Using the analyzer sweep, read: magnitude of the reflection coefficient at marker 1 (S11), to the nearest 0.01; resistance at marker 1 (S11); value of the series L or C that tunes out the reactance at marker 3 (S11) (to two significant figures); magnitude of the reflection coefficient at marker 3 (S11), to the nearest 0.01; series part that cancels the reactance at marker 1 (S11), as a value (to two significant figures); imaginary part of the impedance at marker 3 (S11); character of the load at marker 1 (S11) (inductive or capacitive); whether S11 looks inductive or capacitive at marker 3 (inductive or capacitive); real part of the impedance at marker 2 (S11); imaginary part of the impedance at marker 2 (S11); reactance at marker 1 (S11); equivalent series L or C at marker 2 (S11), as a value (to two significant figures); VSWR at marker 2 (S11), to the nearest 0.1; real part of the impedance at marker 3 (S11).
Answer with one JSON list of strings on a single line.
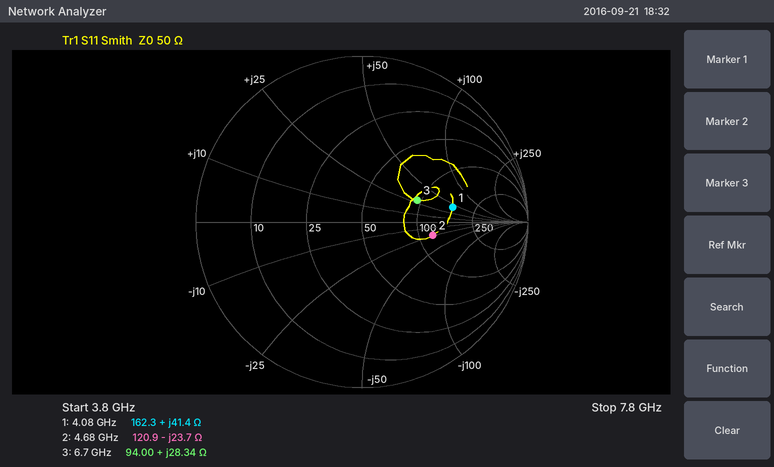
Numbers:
["0.55", "162.3 Ω", "840 fF", "0.36", "940 fF", "+28.34 Ω", "inductive", "inductive", "120.9 Ω", "-23.7 Ω", "+41.4 Ω", "1.4 pF", "2.5", "94.00 Ω"]
